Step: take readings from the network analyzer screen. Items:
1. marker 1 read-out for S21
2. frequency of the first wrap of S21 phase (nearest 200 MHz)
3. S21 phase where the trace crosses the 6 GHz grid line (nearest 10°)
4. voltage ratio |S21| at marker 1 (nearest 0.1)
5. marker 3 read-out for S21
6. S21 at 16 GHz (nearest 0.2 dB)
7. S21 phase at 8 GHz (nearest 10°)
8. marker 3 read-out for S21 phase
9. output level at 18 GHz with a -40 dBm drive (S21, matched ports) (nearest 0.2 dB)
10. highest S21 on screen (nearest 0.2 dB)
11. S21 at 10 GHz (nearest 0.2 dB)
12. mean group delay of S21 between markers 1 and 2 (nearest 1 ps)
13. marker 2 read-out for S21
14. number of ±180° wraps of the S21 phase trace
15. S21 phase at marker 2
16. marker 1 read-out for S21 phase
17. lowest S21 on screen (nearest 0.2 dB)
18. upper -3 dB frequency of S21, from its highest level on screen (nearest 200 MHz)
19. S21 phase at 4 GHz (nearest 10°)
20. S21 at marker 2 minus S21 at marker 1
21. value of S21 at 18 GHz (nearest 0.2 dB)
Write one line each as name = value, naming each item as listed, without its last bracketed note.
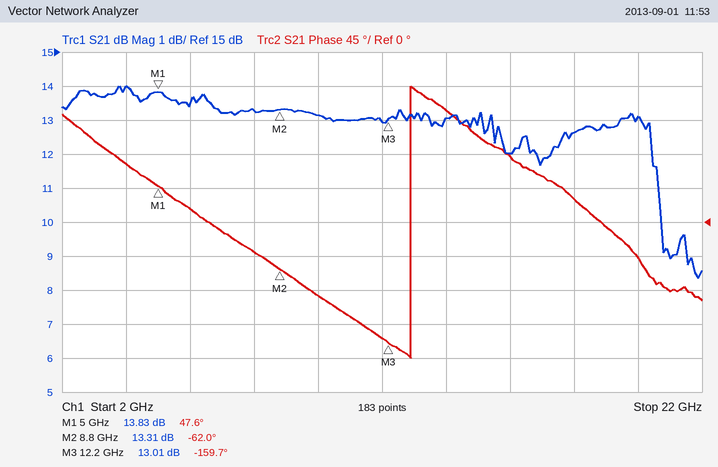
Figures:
marker 1 read-out for S21 = 13.83 dB
frequency of the first wrap of S21 phase = 13.0 GHz
S21 phase where the trace crosses the 6 GHz grid line = 20°
voltage ratio |S21| at marker 1 = 4.9
marker 3 read-out for S21 = 13.01 dB
S21 at 16 GHz = 12.0 dB
S21 phase at 8 GHz = -40°
marker 3 read-out for S21 phase = -159.7°
output level at 18 GHz with a -40 dBm drive (S21, matched ports) = -27.4 dBm
highest S21 on screen = 14.0 dB
S21 at 10 GHz = 13.2 dB
mean group delay of S21 between markers 1 and 2 = 80 ps
marker 2 read-out for S21 = 13.31 dB
number of ±180° wraps of the S21 phase trace = 1
S21 phase at marker 2 = -62.0°
marker 1 read-out for S21 phase = 47.6°
lowest S21 on screen = 8.4 dB
upper -3 dB frequency of S21, from its highest level on screen = 20.6 GHz
S21 phase at 4 GHz = 80°
S21 at marker 2 minus S21 at marker 1 = -0.52 dB
value of S21 at 18 GHz = 12.6 dB
